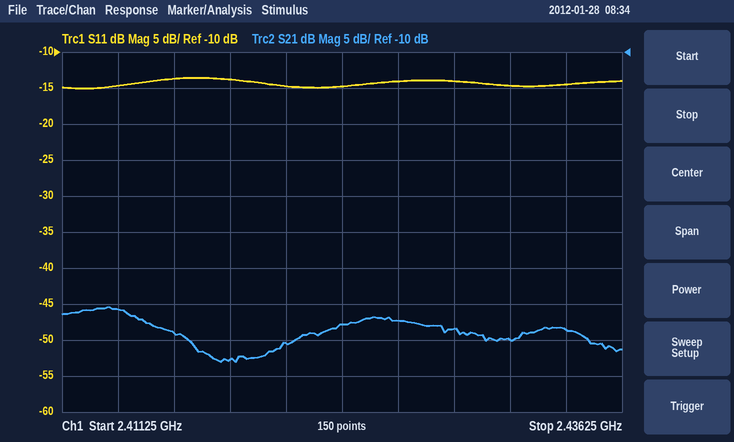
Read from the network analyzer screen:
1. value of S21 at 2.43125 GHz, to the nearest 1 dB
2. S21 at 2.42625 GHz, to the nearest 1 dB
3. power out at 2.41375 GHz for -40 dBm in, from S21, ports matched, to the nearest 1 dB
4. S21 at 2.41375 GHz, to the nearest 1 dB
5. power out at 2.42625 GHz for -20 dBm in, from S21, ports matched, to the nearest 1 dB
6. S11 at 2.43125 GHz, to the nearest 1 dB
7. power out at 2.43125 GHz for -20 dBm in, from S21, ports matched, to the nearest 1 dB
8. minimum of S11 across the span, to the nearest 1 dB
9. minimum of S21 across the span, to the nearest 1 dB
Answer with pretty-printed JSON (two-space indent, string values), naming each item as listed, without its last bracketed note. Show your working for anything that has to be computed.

{
  "value of S21 at 2.43125 GHz, to the nearest 1 dB": "-50 dB",
  "S21 at 2.42625 GHz, to the nearest 1 dB": "-47 dB",
  "power out at 2.41375 GHz for -40 dBm in, from S21, ports matched, to the nearest 1 dB": "-40 dBm + (-46 dB) = -86 dBm",
  "S21 at 2.41375 GHz, to the nearest 1 dB": "-46 dB",
  "power out at 2.42625 GHz for -20 dBm in, from S21, ports matched, to the nearest 1 dB": "-20 dBm + (-47 dB) = -67 dBm",
  "S11 at 2.43125 GHz, to the nearest 1 dB": "-15 dB",
  "power out at 2.43125 GHz for -20 dBm in, from S21, ports matched, to the nearest 1 dB": "-20 dBm + (-50 dB) = -70 dBm",
  "minimum of S11 across the span, to the nearest 1 dB": "-15 dB",
  "minimum of S21 across the span, to the nearest 1 dB": "-53 dB"
}
